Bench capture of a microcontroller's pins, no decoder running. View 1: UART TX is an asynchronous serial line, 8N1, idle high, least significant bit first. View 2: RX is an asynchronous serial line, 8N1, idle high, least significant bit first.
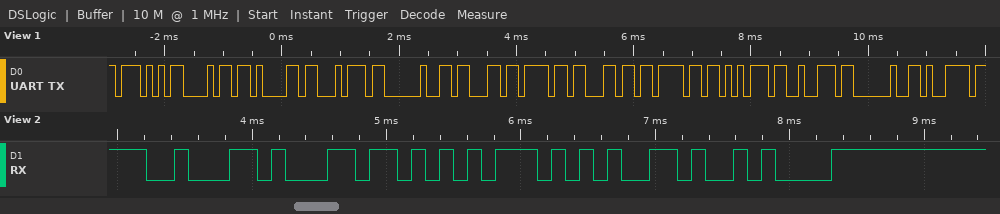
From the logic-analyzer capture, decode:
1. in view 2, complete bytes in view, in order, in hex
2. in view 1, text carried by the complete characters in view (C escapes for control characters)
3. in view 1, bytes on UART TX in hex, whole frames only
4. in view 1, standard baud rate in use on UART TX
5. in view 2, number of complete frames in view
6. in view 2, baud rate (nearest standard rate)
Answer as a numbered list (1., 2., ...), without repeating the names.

1. 62 6C 75 65 0A
2. "What colour y"
3. 57 68 61 74 20 63 6F 6C 6F 75 72 20 79
4. 9600 baud
5. 5
6. 9600 baud
